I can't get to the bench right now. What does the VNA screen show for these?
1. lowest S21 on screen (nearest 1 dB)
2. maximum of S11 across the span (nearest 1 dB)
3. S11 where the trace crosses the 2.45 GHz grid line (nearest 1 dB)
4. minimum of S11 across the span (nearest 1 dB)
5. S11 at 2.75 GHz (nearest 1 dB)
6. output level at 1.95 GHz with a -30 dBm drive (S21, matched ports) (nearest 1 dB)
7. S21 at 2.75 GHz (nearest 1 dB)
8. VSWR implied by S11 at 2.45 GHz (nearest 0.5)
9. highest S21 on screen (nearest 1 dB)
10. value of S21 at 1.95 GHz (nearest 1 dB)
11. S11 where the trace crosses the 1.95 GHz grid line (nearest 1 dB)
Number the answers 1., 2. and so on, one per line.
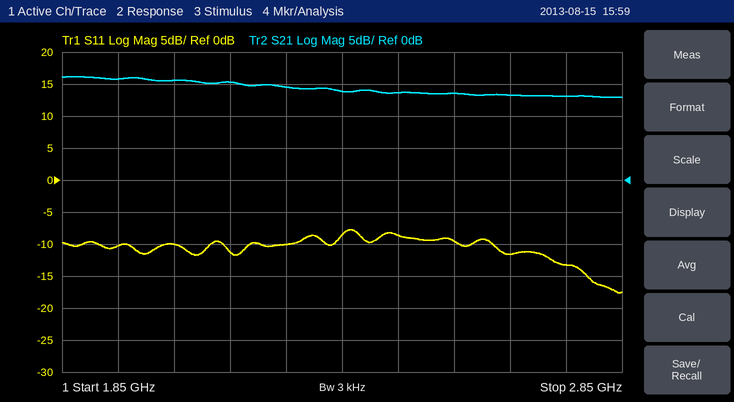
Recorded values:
1. 13 dB
2. -8 dB
3. -9 dB
4. -18 dB
5. -13 dB
6. -14 dBm
7. 13 dB
8. 2.0
9. 16 dB
10. 16 dB
11. -10 dB
